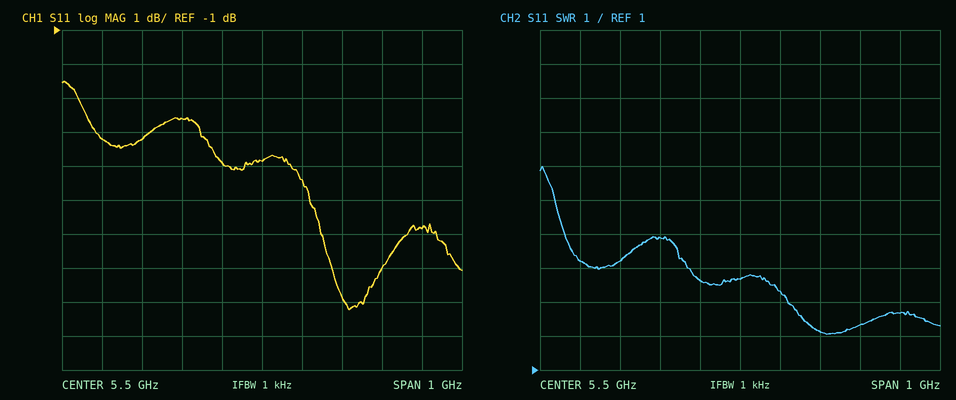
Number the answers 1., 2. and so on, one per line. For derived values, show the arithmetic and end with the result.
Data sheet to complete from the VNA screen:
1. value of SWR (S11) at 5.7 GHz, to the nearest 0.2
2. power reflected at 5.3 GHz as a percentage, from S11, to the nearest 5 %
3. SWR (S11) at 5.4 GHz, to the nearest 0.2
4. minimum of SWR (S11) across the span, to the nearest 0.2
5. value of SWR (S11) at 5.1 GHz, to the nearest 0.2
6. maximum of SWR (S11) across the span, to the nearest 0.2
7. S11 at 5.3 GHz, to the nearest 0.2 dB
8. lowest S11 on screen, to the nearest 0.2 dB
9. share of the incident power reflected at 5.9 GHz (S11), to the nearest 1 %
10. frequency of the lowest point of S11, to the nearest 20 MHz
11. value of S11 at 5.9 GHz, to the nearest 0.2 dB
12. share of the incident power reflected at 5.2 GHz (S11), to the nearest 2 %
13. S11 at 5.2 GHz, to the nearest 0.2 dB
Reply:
1. 2.2
2. 10^(-3.6/10) ≈ 43.7 %, so 45 % to the nearest 5 %
3. 3.6
4. 2.0
5. 4.2
6. 7.0
7. -3.6 dB
8. -9.2 dB
9. 10^(-6.8/10) ≈ 21 %
10. 5.72 GHz
11. -6.8 dB
12. 10^(-4.2/10) ≈ 38 %
13. -4.2 dB
